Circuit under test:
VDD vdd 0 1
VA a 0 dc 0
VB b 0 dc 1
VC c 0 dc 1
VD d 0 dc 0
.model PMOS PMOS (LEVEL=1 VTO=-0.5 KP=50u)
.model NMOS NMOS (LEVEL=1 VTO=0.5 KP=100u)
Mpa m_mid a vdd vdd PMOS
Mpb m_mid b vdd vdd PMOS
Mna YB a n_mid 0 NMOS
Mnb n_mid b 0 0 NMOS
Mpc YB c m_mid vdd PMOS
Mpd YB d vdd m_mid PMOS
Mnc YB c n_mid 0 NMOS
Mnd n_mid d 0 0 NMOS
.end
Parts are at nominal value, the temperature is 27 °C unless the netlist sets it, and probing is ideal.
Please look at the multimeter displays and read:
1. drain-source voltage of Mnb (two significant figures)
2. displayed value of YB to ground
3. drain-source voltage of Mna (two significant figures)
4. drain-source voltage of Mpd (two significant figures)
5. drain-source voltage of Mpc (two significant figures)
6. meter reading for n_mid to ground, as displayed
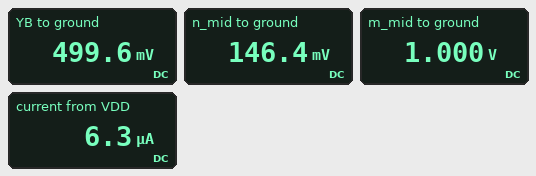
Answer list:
150 mV
499.6 mV
350 mV
-500 mV
-500 mV
146.4 mV
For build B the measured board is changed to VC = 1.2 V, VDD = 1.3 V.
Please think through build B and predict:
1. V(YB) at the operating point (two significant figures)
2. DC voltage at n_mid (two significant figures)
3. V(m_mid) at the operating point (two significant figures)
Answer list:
1.0 V
260 mV
1.3 V
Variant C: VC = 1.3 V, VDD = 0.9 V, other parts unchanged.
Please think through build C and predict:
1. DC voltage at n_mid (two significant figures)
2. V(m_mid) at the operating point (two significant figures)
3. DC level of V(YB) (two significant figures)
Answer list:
88 mV
900 mV
150 mV
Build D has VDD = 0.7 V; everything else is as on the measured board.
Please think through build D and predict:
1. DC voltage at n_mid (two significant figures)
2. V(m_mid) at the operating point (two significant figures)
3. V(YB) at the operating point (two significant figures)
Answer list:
20 mV
700 mV
42 mV
